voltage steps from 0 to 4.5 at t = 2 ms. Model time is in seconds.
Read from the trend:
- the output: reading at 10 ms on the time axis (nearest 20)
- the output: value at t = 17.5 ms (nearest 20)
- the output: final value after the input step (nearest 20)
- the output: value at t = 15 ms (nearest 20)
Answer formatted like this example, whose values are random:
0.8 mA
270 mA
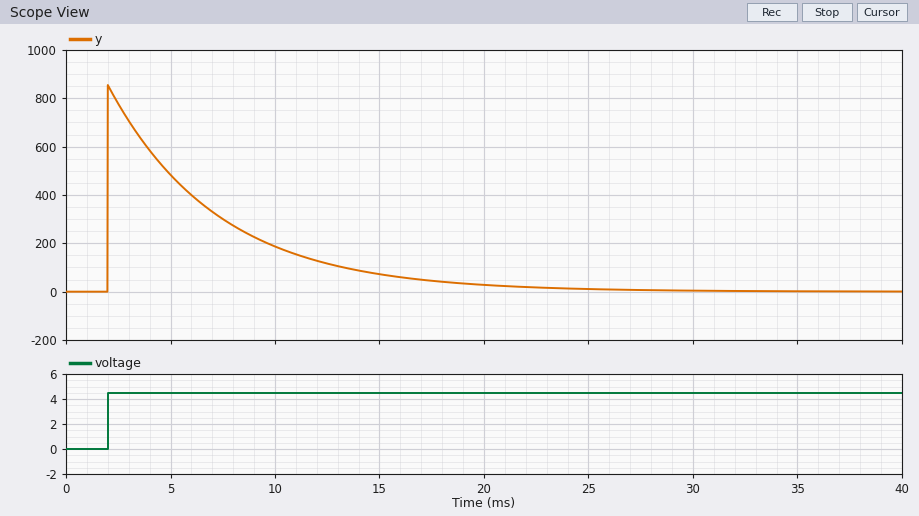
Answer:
180
40
0
80
